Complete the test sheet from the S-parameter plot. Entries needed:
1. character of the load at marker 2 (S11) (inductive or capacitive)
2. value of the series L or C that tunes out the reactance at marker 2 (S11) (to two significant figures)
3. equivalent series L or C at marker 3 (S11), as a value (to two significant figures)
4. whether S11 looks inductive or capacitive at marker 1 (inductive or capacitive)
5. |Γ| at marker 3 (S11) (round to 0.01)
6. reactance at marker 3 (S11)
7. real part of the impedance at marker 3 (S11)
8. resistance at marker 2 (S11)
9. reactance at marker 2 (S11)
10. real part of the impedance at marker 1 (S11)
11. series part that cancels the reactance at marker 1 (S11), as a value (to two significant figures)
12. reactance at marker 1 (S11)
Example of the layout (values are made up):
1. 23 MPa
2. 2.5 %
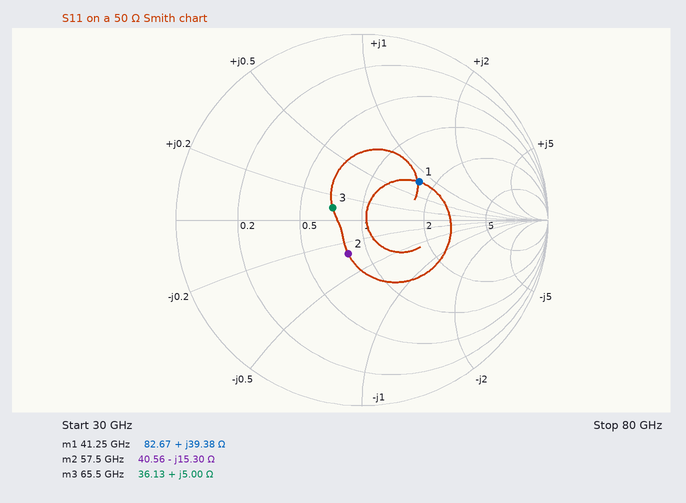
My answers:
1. capacitive
2. 42 pH
3. 12 pH
4. inductive
5. 0.17
6. +5.00 Ω
7. 36.13 Ω
8. 40.56 Ω
9. -15.30 Ω
10. 82.67 Ω
11. 98 fF
12. +39.38 Ω
